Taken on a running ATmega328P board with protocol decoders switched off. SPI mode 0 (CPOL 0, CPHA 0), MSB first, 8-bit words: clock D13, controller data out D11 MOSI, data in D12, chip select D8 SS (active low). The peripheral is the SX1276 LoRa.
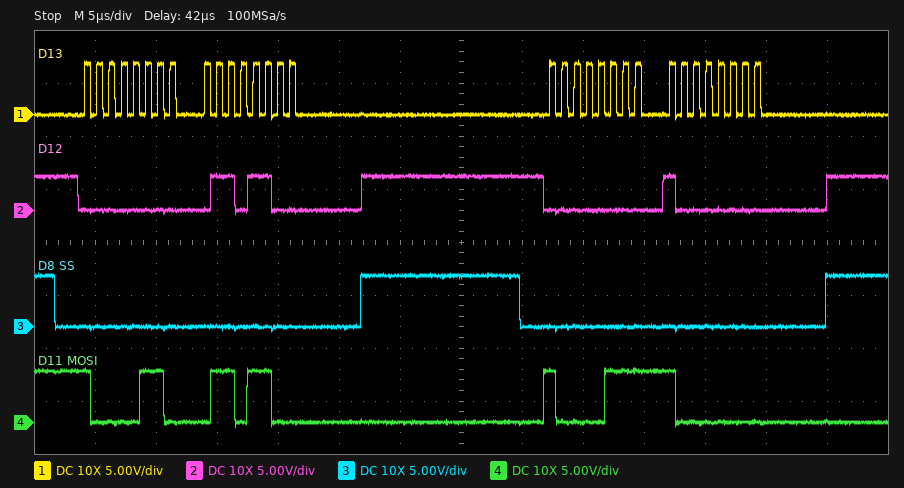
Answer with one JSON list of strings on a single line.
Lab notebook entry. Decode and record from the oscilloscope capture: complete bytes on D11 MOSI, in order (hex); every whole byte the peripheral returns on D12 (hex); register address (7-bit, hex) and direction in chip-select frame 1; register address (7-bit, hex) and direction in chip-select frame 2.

["86 6C 87 80", "00 6C 00 80", "0x06 write", "0x07 write"]
